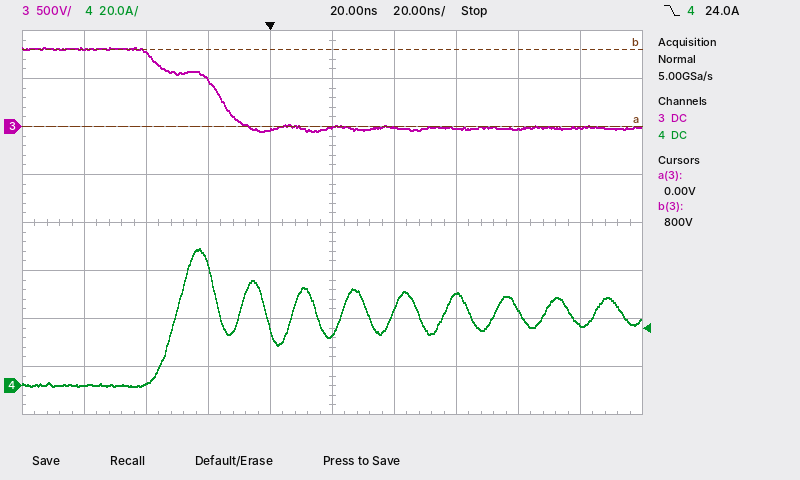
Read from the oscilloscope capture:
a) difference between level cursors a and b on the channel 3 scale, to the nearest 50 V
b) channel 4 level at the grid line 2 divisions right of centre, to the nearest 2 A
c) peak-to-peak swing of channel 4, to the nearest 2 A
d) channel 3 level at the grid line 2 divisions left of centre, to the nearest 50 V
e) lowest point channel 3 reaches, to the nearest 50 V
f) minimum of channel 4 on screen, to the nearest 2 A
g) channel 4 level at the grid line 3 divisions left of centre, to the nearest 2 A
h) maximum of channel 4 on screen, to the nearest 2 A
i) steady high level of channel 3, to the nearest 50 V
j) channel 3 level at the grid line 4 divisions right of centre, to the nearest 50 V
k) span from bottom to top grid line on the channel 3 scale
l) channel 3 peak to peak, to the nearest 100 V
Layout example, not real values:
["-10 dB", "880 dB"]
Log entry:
["800 V", "38 A", "58 A", "500 V", "-50 V", "0 A", "0 A", "58 A", "800 V", "0 V", "4 kV", "900 V"]
